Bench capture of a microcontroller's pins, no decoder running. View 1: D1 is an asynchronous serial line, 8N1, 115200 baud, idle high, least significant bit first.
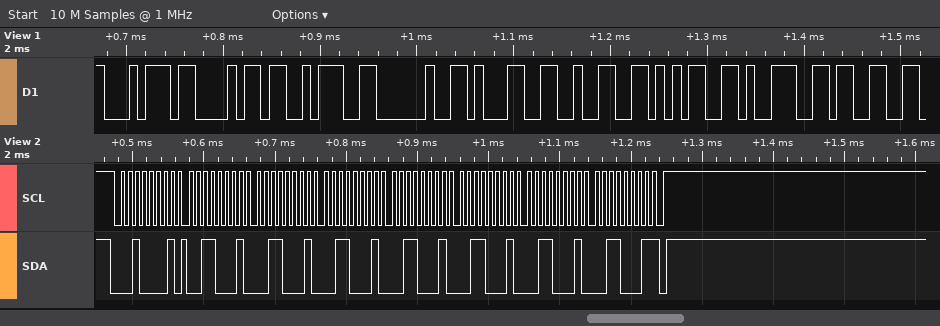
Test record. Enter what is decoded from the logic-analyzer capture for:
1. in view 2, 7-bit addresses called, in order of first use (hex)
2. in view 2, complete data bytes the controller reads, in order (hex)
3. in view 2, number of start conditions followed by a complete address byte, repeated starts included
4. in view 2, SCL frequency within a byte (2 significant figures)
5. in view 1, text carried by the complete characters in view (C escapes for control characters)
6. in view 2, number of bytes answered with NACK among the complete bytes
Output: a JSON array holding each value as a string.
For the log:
["0x10", "31 31 31 31 31 31 31", "1", "100 kHz", "\"th: 12593\"", "1"]
